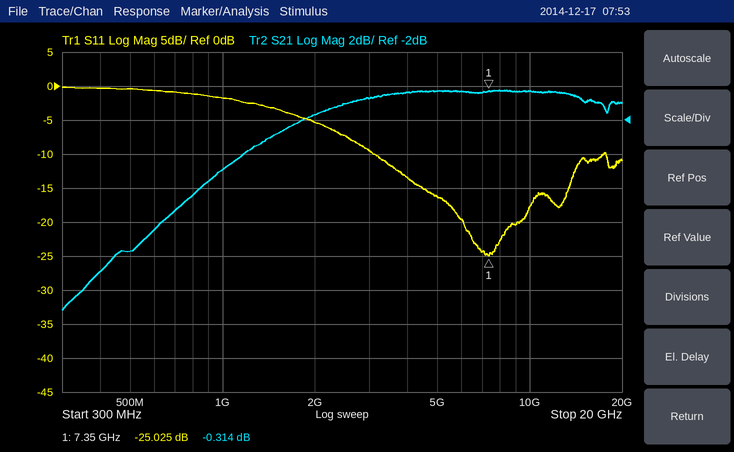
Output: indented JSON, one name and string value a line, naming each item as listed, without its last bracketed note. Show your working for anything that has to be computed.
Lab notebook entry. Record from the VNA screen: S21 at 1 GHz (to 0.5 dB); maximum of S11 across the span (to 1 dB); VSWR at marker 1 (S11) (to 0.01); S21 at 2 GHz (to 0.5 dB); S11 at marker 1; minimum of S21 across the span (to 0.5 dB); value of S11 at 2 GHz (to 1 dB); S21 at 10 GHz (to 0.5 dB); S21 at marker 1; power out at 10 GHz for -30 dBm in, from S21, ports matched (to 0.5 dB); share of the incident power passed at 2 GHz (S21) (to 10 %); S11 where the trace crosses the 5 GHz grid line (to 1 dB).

{
  "S21 at 1 GHz": "-5.0 dB",
  "maximum of S11 across the span": "0 dB",
  "VSWR at marker 1 (S11)": "(1 + 0.0561)/(1 − 0.0561) ≈ 1.12",
  "S21 at 2 GHz": "-1.5 dB",
  "S11 at marker 1": "-25.025 dB",
  "minimum of S21 across the span": "-13.0 dB",
  "value of S11 at 2 GHz": "-5 dB",
  "S21 at 10 GHz": "-0.5 dB",
  "S21 at marker 1": "-0.314 dB",
  "power out at 10 GHz for -30 dBm in, from S21, ports matched": "-30 dBm + (-0.5 dB) = -30.5 dBm",
  "share of the incident power passed at 2 GHz (S21)": "10^(-1.5/10) ≈ 70.8 %, so 70 % to the nearest 10 %",
  "S11 where the trace crosses the 5 GHz grid line": "-16 dB"
}
